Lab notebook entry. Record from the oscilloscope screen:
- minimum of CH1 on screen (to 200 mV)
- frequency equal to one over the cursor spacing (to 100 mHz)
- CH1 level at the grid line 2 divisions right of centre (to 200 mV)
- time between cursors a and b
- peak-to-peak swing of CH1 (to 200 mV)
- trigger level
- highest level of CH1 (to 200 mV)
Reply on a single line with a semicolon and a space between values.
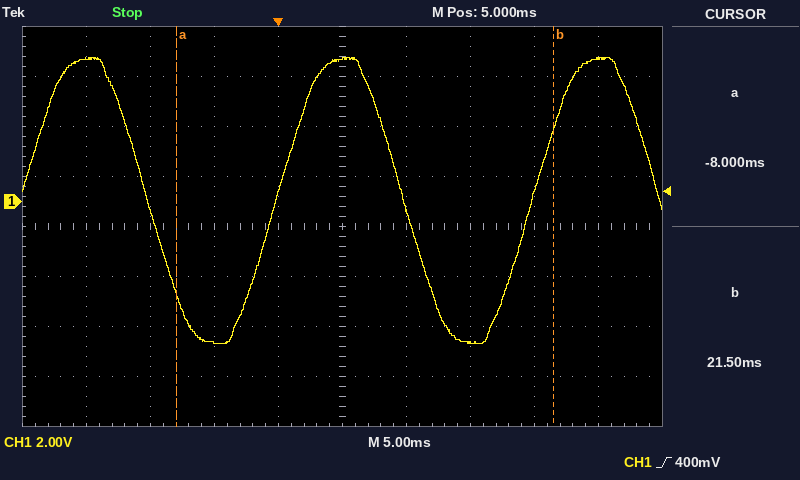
-5.6 V; 33.9 Hz; -5.6 V; 29.5 ms; 11.4 V; 400 mV; 5.8 V
